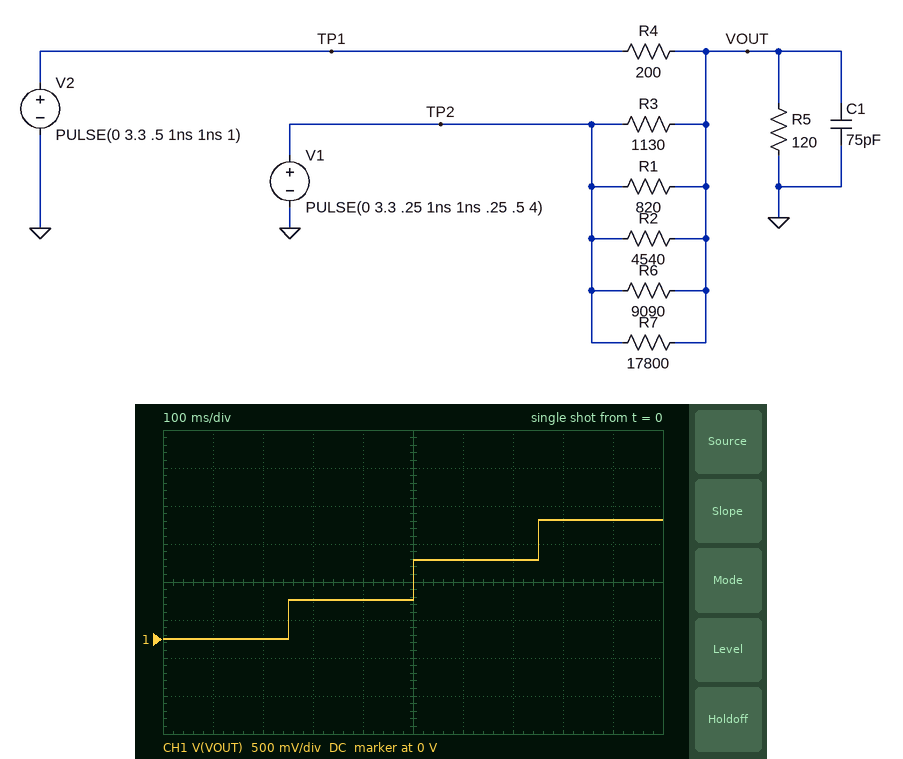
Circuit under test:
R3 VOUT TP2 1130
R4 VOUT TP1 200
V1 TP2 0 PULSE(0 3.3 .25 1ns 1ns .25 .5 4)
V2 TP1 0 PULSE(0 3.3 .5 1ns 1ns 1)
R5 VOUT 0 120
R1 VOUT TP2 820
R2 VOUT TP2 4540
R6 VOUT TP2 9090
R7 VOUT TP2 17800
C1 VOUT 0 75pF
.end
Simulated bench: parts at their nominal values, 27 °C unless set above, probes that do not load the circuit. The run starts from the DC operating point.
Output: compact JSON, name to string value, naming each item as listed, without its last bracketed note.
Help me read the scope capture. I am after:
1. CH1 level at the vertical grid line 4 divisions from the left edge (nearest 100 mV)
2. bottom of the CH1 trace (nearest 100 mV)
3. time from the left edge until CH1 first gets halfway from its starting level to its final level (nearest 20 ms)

{"CH1 level at the vertical grid line 4 divisions from the left edge": "500 mV", "bottom of the CH1 trace": "0 V", "time from the left edge until CH1 first gets halfway from its starting level to its final level": "500 ms"}
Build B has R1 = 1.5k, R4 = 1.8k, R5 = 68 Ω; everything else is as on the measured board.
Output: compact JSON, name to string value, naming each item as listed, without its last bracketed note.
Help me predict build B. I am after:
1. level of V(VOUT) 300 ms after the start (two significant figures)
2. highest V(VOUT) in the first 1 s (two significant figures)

{"level of V(VOUT) 300 ms after the start": "370 mV", "highest V(VOUT) in the first 1 s": "480 mV"}
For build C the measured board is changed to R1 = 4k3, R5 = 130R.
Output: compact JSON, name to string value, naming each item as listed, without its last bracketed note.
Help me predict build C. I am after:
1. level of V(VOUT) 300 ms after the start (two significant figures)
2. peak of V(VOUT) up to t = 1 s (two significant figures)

{"level of V(VOUT) 300 ms after the start": "350 mV", "peak of V(VOUT) up to t = 1 s": "1.5 V"}
